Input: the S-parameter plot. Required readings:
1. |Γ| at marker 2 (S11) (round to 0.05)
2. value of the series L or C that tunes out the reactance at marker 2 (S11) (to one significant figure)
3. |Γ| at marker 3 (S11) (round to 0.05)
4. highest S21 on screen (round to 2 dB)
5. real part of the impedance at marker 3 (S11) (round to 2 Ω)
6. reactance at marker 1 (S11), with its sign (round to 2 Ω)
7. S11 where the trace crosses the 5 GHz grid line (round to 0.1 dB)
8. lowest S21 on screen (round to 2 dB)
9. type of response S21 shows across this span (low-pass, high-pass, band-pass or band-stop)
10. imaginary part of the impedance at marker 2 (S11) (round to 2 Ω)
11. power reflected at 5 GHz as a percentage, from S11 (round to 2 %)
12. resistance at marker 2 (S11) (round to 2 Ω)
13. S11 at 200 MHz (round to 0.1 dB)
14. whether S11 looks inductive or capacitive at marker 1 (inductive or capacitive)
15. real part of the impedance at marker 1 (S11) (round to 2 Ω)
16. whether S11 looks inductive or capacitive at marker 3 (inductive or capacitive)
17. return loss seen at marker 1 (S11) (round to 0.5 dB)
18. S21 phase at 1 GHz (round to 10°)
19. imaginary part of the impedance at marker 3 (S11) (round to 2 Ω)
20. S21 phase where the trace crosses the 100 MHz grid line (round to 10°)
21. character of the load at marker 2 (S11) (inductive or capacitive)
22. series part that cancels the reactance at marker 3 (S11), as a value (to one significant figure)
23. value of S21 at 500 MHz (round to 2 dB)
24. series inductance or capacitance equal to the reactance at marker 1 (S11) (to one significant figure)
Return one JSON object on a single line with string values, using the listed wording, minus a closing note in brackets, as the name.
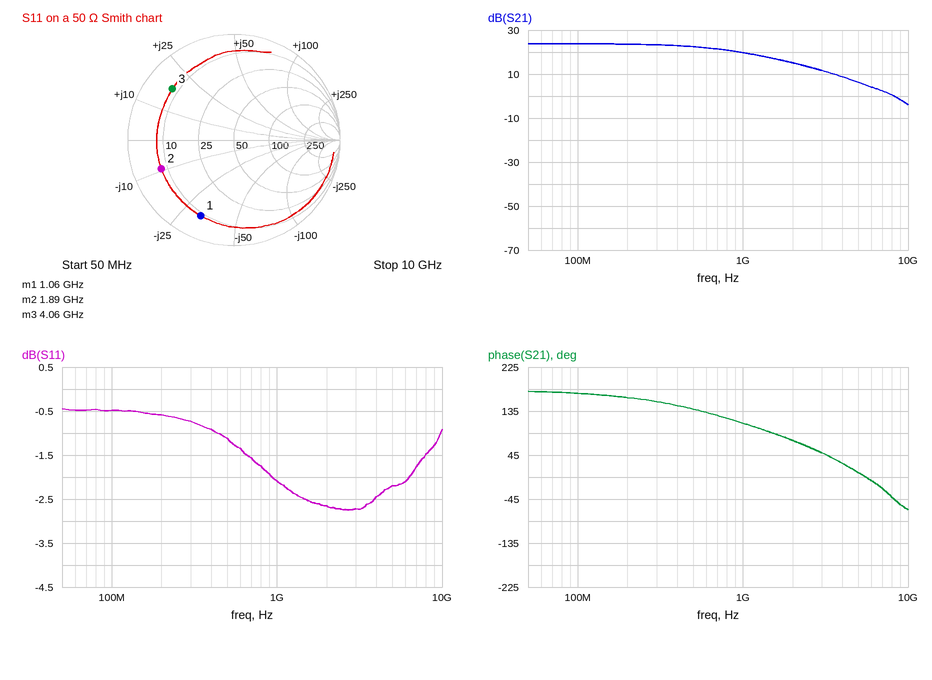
{"|Γ| at marker 2 (S11)": "0.75", "value of the series L or C that tunes out the reactance at marker 2 (S11)": "800 pH", "|Γ| at marker 3 (S11)": "0.75", "highest S21 on screen": "24 dB", "real part of the impedance at marker 3 (S11)": "8 Ω", "reactance at marker 1 (S11), with its sign": "-32 Ω", "S11 where the trace crosses the 5 GHz grid line": "-2.2 dB", "lowest S21 on screen": "-4 dB", "type of response S21 shows across this span": "low-pass", "imaginary part of the impedance at marker 2 (S11)": "-10 Ω", "power reflected at 5 GHz as a percentage, from S11": "60 %", "resistance at marker 2 (S11)": "8 Ω", "S11 at 200 MHz": "-0.6 dB", "whether S11 looks inductive or capacitive at marker 1": "capacitive", "real part of the impedance at marker 1 (S11)": "8 Ω", "whether S11 looks inductive or capacitive at marker 3": "inductive", "return loss seen at marker 1 (S11)": "2.0 dB", "S21 phase at 1 GHz": "110°", "imaginary part of the impedance at marker 3 (S11)": "+18 Ω", "S21 phase where the trace crosses the 100 MHz grid line": "170°", "character of the load at marker 2 (S11)": "capacitive", "series part that cancels the reactance at marker 3 (S11), as a value": "2 pF", "value of S21 at 500 MHz": "22 dB", "series inductance or capacitance equal to the reactance at marker 1 (S11)": "5 pF"}
